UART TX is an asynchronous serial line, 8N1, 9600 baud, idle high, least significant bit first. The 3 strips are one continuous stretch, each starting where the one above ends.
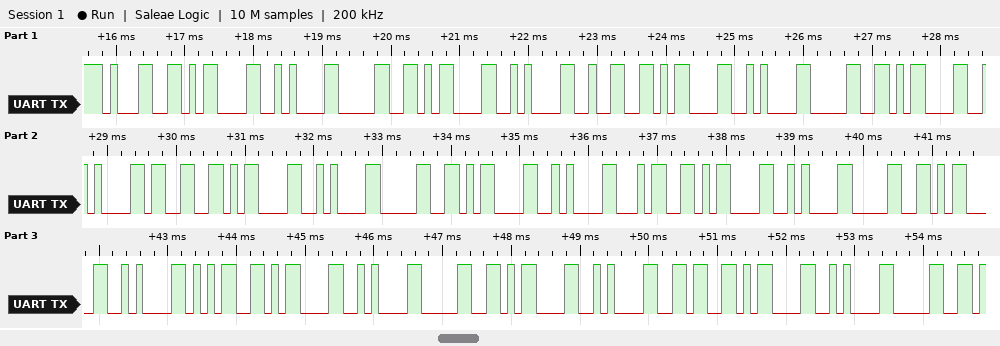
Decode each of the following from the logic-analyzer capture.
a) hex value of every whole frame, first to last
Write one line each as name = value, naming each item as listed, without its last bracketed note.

hex value of every whole frame, first to last = 31 0D 0A 30 0D 0A 32 0D 0A 30 0D 0A 33 0D 0A 30 0D 0A 34 0D 0A 30 0D 0A 35 0D 0A 30 0D 0A 36 0D 0A 30
